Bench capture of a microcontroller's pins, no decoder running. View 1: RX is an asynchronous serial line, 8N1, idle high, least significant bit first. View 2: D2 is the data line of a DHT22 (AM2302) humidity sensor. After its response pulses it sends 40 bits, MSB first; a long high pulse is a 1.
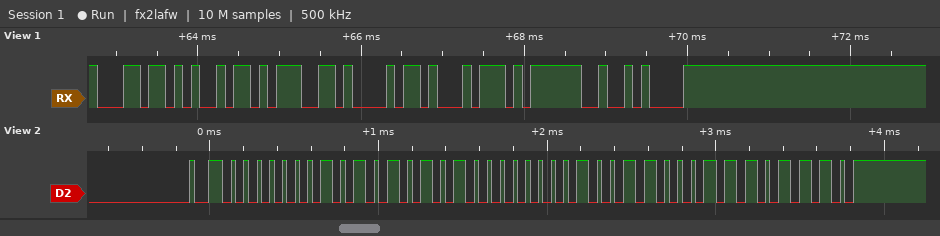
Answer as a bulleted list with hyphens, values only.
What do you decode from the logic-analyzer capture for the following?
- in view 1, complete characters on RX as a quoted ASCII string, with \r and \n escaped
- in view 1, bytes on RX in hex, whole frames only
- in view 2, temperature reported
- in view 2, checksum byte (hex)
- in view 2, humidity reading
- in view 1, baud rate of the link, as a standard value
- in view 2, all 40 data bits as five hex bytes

- "light?\n"
- 6C 69 67 68 74 3F 0A
- 15.2 °C
- 0xEE
- 34.1 %
- 9600 baud
- 01 55 00 98 EE
